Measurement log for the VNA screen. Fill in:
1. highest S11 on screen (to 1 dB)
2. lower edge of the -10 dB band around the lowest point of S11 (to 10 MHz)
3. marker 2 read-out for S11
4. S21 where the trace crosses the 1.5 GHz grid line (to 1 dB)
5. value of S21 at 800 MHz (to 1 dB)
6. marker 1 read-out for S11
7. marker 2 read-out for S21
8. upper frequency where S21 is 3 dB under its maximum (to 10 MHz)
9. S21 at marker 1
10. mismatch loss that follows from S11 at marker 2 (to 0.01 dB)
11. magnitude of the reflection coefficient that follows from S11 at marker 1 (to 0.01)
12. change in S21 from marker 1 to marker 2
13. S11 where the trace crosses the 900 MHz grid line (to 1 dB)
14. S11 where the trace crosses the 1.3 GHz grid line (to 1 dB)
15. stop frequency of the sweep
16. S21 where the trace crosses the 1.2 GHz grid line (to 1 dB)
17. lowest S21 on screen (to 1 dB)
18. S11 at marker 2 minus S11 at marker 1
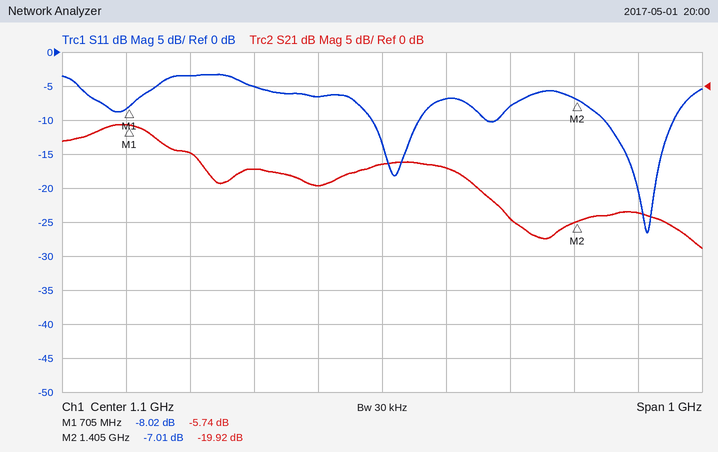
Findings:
-3 dB
1.45 GHz
-7.01 dB
-19 dB
-10 dB
-8.02 dB
-19.92 dB
760 MHz
-5.74 dB
0.96 dB
0.40
-14.18 dB
-5 dB
-8 dB
1.6 GHz
-12 dB
-24 dB
1.01 dB
